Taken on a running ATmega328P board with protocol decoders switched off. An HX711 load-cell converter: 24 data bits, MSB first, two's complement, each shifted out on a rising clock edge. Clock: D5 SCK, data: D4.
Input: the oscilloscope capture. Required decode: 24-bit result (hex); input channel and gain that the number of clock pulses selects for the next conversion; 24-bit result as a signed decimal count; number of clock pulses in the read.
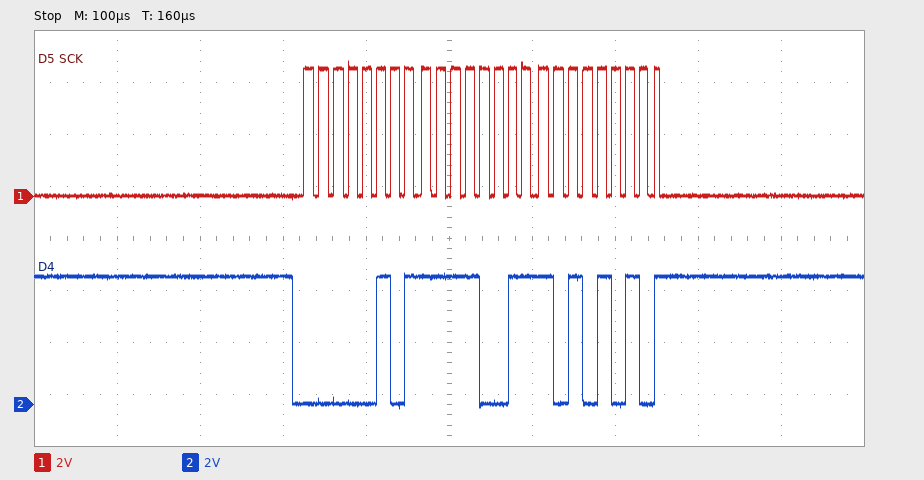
0x05F3AA
channel A, gain 128
390058
25
